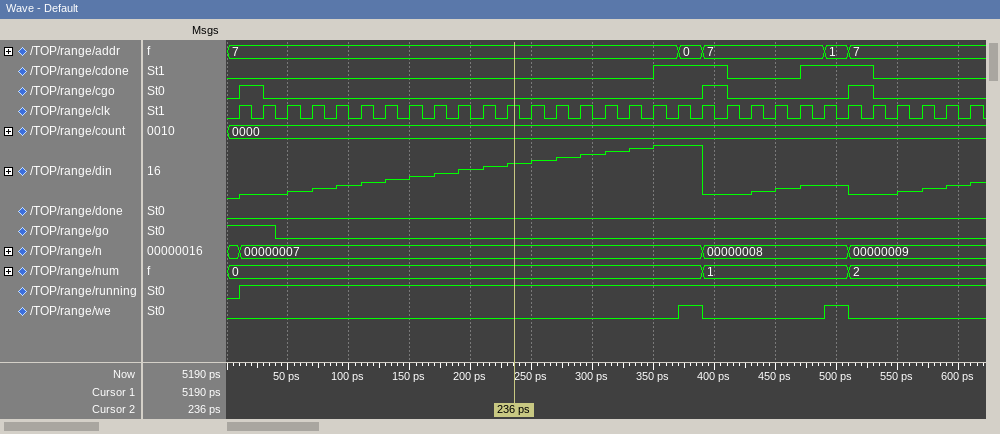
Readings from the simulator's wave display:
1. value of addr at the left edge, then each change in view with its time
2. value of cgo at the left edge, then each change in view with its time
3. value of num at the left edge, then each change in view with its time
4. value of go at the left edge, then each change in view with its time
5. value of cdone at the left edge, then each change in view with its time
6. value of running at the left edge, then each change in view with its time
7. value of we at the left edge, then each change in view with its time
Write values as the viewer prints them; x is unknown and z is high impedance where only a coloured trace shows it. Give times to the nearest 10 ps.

7, 0 at 370 ps, 7 at 390 ps, 1 at 490 ps, 7 at 510 ps
0, 1 at 10 ps, 0 at 30 ps, 1 at 390 ps, 0 at 410 ps, 1 at 510 ps, 0 at 530 ps
0, 1 at 390 ps, 2 at 510 ps
1, 0 at 40 ps
0, 1 at 350 ps, 0 at 410 ps, 1 at 470 ps, 0 at 530 ps
0, 1 at 10 ps
0, 1 at 370 ps, 0 at 390 ps, 1 at 490 ps, 0 at 510 ps
